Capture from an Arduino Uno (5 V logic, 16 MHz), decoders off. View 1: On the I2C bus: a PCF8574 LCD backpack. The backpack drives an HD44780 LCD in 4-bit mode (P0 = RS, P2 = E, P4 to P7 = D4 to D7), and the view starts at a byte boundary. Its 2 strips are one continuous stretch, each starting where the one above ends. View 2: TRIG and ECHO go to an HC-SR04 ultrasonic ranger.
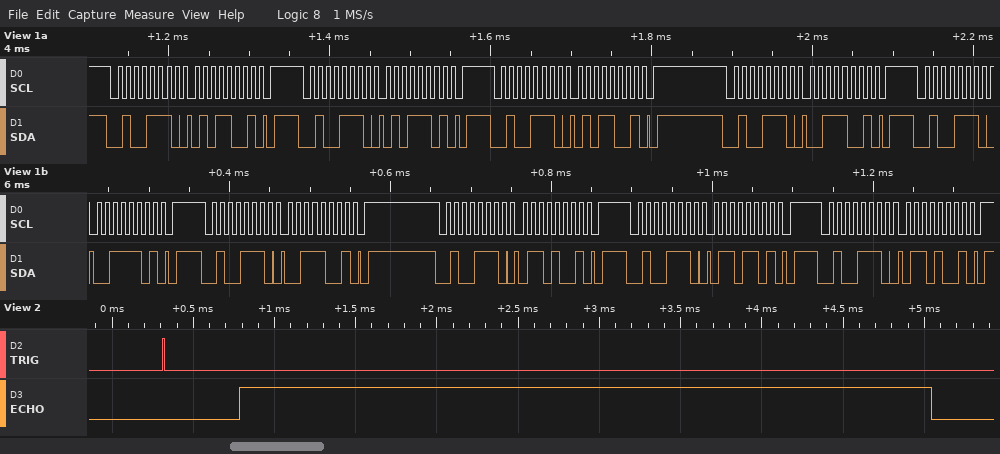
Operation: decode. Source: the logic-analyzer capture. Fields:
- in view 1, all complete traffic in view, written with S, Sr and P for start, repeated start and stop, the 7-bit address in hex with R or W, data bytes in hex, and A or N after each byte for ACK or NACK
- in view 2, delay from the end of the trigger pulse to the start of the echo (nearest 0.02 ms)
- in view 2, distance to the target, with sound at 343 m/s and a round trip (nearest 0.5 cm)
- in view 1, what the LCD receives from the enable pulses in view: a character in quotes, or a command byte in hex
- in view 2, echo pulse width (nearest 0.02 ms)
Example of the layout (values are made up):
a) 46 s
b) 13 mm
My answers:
a) S 27W A 59 A P S 27W A 5D A P S 27W A 59 A P S 27W A 39 A P S 27W A 3D A P S 27W A 39 A P S 27W A 69 A P S 27W A 6D A P S 27W A 69 A P
b) 0.46 ms
c) 73 cm
d) 'S'
e) 4.26 ms
